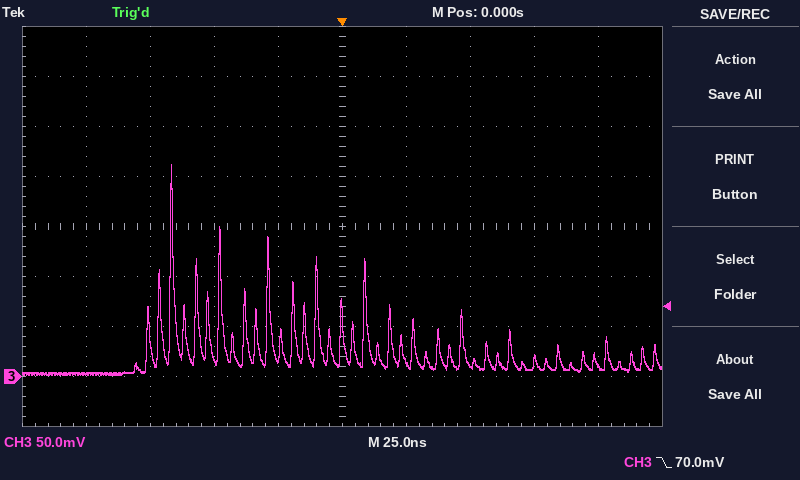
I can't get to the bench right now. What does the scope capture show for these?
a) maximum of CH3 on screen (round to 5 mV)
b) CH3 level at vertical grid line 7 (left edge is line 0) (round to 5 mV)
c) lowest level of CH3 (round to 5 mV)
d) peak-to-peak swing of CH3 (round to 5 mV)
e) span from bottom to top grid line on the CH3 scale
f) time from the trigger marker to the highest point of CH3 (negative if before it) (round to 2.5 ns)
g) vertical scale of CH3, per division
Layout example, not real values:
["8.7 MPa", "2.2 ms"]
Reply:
["210 mV", "10 mV", "0 mV", "210 mV", "400 mV", "-67.5 ns", "50 mV"]
